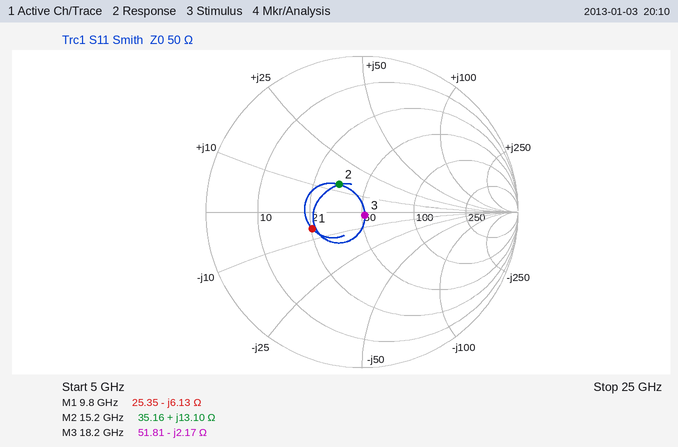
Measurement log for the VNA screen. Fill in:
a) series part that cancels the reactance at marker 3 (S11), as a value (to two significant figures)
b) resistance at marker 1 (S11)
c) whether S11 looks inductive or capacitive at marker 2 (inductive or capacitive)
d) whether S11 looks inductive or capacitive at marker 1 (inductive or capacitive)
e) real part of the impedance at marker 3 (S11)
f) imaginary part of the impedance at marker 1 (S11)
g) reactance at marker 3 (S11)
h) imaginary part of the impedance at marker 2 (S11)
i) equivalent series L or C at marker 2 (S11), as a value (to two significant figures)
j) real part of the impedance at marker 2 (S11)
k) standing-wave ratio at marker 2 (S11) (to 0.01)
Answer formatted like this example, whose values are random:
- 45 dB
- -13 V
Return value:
- 19 pH
- 25.35 Ω
- inductive
- capacitive
- 51.81 Ω
- -6.13 Ω
- -2.17 Ω
- +13.10 Ω
- 140 pH
- 35.16 Ω
- 1.60
